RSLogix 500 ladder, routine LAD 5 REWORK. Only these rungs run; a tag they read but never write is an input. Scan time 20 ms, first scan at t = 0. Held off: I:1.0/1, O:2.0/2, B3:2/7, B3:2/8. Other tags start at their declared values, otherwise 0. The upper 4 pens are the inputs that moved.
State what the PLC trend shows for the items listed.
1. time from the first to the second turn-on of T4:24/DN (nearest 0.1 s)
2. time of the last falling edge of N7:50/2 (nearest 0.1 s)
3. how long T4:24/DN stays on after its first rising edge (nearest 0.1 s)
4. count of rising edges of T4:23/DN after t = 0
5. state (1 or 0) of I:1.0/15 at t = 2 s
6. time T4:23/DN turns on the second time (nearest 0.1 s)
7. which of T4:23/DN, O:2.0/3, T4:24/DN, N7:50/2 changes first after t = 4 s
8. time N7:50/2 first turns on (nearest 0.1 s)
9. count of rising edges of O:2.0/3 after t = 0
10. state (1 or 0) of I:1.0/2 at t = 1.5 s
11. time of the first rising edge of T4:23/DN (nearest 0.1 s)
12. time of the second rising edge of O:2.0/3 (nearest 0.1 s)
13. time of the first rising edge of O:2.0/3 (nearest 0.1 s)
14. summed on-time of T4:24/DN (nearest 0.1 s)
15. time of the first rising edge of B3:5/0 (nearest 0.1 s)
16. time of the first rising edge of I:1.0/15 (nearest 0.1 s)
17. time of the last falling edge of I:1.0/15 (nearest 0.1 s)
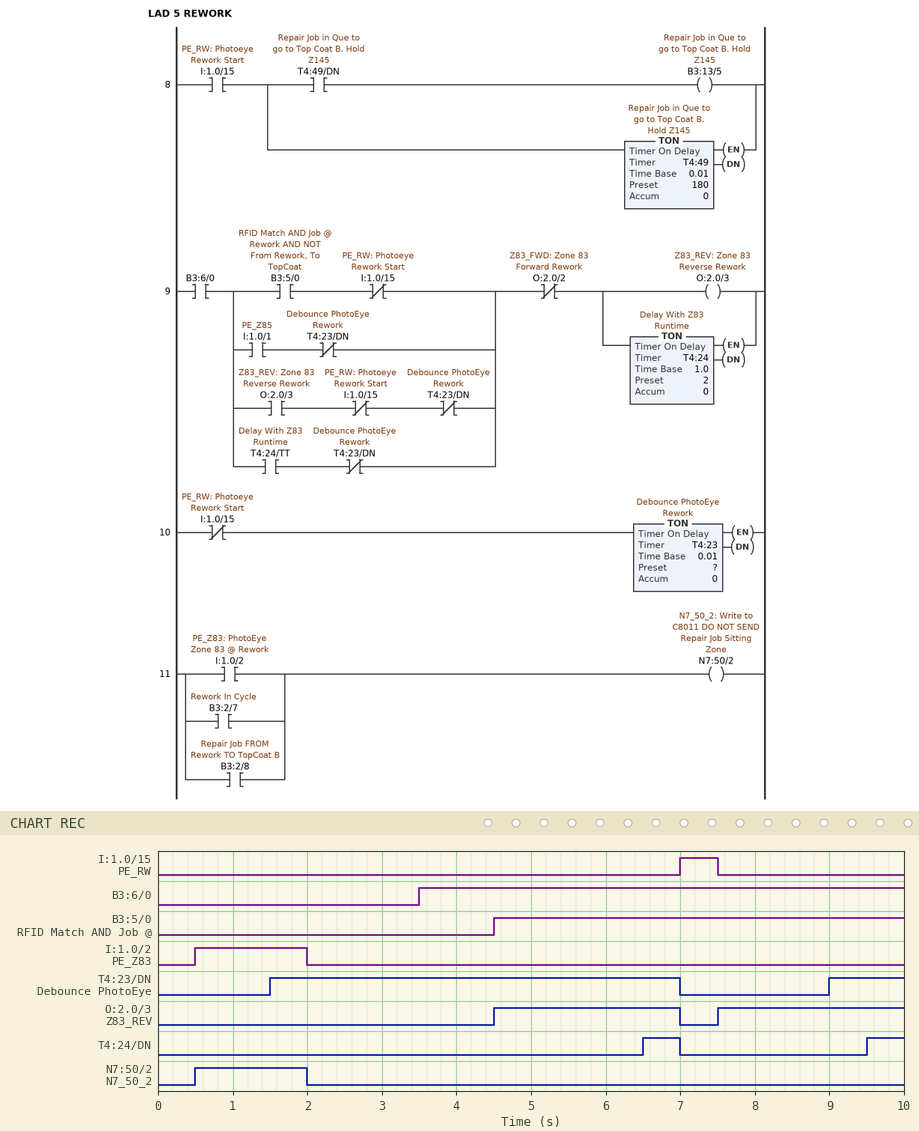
3.0 s
2.0 s
0.5 s
2
0
9.0 s
O:2.0/3
0.5 s
2
1
1.5 s
7.5 s
4.5 s
1.0 s
4.5 s
7.0 s
7.5 s
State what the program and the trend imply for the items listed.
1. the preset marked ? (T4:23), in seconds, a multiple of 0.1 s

1.5 s
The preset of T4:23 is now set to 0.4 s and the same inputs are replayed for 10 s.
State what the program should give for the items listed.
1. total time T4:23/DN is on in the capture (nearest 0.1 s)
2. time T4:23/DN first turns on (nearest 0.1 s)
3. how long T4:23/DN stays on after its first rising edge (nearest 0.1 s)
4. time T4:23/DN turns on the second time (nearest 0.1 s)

8.7 s
0.4 s
6.6 s
7.9 s
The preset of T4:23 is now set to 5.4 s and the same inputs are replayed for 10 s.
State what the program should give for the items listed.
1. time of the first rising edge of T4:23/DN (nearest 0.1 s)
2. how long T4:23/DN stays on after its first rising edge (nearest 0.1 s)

5.4 s
1.6 s
